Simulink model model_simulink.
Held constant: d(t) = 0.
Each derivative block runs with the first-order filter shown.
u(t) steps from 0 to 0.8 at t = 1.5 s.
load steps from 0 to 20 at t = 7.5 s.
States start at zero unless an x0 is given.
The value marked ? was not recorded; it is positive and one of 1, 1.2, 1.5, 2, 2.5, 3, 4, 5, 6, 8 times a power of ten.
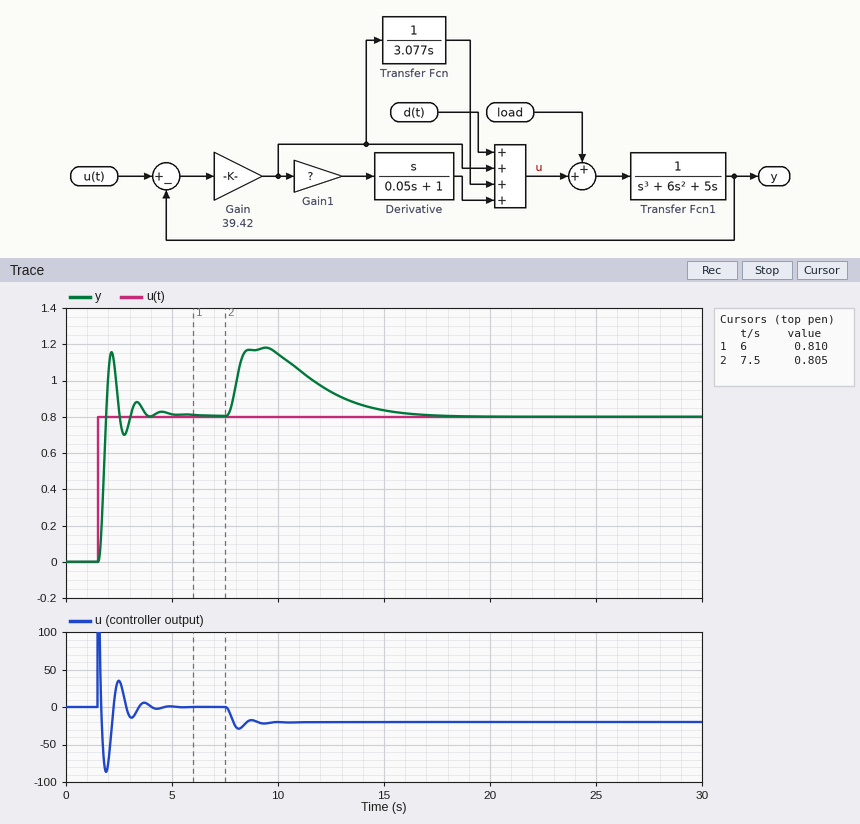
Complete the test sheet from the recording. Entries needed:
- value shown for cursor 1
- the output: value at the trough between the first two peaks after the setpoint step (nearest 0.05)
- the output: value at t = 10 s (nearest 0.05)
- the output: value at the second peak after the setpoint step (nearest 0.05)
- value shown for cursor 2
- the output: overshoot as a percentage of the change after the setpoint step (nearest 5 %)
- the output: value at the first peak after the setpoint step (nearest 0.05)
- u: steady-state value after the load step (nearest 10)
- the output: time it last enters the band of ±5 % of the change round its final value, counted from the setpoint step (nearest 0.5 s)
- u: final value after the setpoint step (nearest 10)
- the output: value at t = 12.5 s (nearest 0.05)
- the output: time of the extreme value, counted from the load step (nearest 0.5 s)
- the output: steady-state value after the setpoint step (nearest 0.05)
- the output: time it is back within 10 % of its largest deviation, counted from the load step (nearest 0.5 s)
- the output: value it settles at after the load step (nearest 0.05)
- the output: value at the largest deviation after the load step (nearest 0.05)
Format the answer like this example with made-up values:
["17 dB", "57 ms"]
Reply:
["0.810", "0.70", "1.15", "0.90", "0.805", "45 %", "1.15", "-20", "2.0 s", "0", "0.95", "2.0 s", "0.80", "7.5 s", "0.80", "1.20"]
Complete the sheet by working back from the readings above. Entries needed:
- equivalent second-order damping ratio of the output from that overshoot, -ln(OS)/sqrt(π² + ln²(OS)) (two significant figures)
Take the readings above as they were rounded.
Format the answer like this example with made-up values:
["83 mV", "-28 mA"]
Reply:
["0.25"]
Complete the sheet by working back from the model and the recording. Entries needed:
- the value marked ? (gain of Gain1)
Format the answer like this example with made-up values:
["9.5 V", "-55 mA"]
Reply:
["0.8"]
